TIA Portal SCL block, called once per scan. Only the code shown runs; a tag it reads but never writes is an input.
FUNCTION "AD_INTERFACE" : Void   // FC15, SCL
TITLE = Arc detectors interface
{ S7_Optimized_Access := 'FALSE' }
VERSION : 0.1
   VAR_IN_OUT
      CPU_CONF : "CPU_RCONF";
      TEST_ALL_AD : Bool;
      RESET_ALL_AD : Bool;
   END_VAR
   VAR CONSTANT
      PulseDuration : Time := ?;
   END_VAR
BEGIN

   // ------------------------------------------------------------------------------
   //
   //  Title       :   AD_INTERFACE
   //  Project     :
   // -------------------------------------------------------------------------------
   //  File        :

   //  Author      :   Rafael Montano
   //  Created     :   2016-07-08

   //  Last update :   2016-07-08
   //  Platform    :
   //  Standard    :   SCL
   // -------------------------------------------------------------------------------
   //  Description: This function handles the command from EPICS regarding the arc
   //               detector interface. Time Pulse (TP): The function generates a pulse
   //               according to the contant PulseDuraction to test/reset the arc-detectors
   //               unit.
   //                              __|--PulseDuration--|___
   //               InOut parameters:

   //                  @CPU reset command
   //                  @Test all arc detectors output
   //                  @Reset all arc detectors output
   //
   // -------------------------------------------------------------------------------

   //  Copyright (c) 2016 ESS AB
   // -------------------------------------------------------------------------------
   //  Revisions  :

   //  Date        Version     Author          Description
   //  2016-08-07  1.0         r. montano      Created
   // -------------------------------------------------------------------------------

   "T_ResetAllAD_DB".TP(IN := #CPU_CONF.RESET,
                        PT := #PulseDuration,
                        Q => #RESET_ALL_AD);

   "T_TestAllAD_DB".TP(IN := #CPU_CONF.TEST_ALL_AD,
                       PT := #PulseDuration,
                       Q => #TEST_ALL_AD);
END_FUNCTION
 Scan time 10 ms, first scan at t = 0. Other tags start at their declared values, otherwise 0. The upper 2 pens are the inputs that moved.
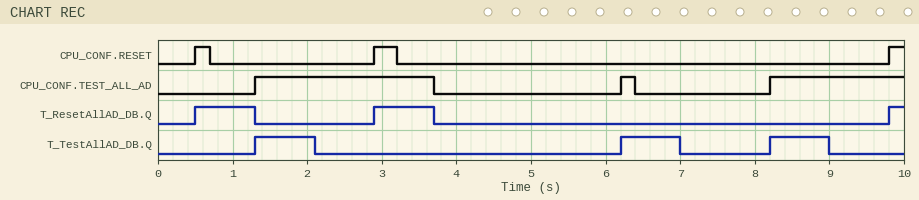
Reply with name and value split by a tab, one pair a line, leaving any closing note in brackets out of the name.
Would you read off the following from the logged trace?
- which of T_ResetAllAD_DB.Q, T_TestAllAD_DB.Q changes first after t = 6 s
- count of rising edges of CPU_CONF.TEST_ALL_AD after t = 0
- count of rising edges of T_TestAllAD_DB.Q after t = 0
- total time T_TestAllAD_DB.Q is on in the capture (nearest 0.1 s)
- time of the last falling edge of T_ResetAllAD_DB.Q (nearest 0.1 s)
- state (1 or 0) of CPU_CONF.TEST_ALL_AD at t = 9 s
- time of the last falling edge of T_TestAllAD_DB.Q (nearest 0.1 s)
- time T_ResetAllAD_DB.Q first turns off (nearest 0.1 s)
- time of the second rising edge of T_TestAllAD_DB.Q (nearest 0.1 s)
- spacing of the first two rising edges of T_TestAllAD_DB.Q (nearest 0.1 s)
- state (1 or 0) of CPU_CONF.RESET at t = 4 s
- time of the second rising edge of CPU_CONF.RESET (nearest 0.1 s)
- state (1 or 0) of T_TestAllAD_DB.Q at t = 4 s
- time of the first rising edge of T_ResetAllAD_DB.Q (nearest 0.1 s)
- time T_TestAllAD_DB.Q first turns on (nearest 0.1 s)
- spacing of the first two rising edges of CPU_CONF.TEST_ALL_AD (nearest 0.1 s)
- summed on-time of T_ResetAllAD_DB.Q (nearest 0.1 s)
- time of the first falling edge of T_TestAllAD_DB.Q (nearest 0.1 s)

which of T_ResetAllAD_DB.Q, T_TestAllAD_DB.Q changes first after t = 6 s	T_TestAllAD_DB.Q
count of rising edges of CPU_CONF.TEST_ALL_AD after t = 0	3
count of rising edges of T_TestAllAD_DB.Q after t = 0	3
total time T_TestAllAD_DB.Q is on in the capture	2.4 s
time of the last falling edge of T_ResetAllAD_DB.Q	3.7 s
state (1 or 0) of CPU_CONF.TEST_ALL_AD at t = 9 s	1
time of the last falling edge of T_TestAllAD_DB.Q	9.0 s
time T_ResetAllAD_DB.Q first turns off	1.3 s
time of the second rising edge of T_TestAllAD_DB.Q	6.2 s
spacing of the first two rising edges of T_TestAllAD_DB.Q	4.9 s
state (1 or 0) of CPU_CONF.RESET at t = 4 s	0
time of the second rising edge of CPU_CONF.RESET	2.9 s
state (1 or 0) of T_TestAllAD_DB.Q at t = 4 s	0
time of the first rising edge of T_ResetAllAD_DB.Q	0.5 s
time T_TestAllAD_DB.Q first turns on	1.3 s
spacing of the first two rising edges of CPU_CONF.TEST_ALL_AD	4.9 s
summed on-time of T_ResetAllAD_DB.Q	1.8 s
time of the first falling edge of T_TestAllAD_DB.Q	2.1 s
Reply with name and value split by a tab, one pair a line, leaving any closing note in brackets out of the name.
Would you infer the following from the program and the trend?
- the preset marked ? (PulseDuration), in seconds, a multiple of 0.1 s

the preset marked ? (PulseDuration), in seconds, a multiple of 0.1 s	0.8 s
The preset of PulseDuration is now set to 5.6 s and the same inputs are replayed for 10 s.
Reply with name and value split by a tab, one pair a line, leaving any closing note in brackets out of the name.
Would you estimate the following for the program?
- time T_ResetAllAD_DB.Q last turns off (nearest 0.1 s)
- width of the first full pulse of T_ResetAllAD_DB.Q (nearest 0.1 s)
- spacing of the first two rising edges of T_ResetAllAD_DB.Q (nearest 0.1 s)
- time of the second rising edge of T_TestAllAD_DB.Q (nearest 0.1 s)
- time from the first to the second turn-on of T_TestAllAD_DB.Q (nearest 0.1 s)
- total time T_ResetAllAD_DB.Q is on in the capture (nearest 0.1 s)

time T_ResetAllAD_DB.Q last turns off	6.1 s
width of the first full pulse of T_ResetAllAD_DB.Q	5.6 s
spacing of the first two rising edges of T_ResetAllAD_DB.Q	9.3 s
time of the second rising edge of T_TestAllAD_DB.Q	8.2 s
time from the first to the second turn-on of T_TestAllAD_DB.Q	6.9 s
total time T_ResetAllAD_DB.Q is on in the capture	5.8 s
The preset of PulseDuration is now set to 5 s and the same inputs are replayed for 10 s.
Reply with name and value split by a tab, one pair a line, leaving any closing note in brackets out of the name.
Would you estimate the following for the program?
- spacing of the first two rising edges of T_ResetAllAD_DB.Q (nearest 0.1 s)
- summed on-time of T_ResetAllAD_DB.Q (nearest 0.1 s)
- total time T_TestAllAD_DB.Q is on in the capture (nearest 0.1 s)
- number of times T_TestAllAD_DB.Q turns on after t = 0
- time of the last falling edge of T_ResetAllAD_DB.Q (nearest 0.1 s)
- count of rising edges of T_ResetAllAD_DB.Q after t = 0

spacing of the first two rising edges of T_ResetAllAD_DB.Q	9.3 s
summed on-time of T_ResetAllAD_DB.Q	5.2 s
total time T_TestAllAD_DB.Q is on in the capture	6.8 s
number of times T_TestAllAD_DB.Q turns on after t = 0	2
time of the last falling edge of T_ResetAllAD_DB.Q	5.5 s
count of rising edges of T_ResetAllAD_DB.Q after t = 0	2
